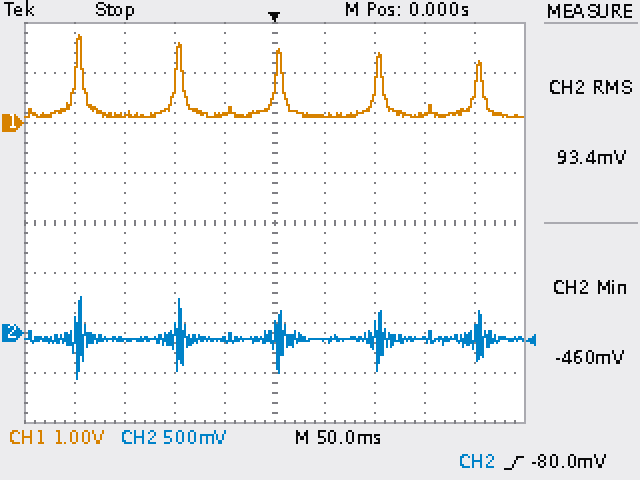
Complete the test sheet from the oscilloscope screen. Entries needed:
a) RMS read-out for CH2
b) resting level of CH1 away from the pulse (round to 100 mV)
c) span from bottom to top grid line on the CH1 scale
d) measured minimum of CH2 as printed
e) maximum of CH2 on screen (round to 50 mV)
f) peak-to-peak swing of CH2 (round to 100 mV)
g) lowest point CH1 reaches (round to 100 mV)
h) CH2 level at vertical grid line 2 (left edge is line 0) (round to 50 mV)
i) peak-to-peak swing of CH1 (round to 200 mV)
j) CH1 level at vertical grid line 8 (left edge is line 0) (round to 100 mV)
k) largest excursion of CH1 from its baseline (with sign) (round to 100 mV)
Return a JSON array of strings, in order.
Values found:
["93.4 mV", "200 mV", "8 V", "-460 mV", "350 mV", "800 mV", "100 mV", "-50 mV", "1.6 V", "200 mV", "+1.6 V"]
